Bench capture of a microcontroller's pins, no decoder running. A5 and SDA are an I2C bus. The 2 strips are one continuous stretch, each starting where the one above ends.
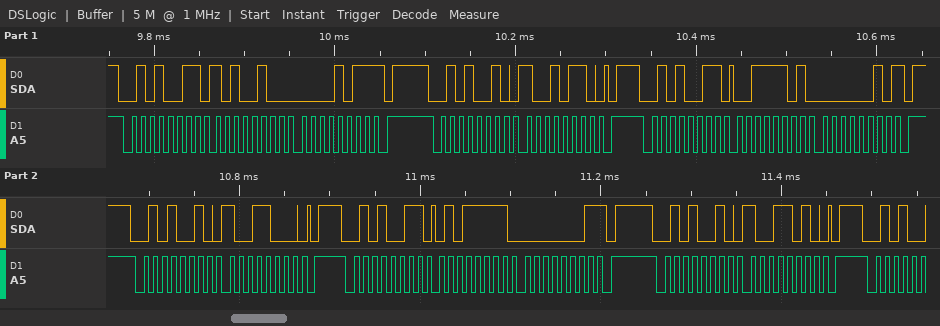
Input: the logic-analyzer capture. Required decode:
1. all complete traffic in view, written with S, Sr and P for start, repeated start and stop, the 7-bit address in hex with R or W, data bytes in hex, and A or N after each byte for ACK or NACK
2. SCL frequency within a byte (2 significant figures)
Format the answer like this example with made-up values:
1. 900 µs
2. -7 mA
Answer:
1. S 29R A A4 A 0B N P S 29W A 96 A P S 29R A 3D A 02 N P S 29W A 98 A P S 29R A 5F A 01 N P S 29W A 9A A P
2. 100 kHz
